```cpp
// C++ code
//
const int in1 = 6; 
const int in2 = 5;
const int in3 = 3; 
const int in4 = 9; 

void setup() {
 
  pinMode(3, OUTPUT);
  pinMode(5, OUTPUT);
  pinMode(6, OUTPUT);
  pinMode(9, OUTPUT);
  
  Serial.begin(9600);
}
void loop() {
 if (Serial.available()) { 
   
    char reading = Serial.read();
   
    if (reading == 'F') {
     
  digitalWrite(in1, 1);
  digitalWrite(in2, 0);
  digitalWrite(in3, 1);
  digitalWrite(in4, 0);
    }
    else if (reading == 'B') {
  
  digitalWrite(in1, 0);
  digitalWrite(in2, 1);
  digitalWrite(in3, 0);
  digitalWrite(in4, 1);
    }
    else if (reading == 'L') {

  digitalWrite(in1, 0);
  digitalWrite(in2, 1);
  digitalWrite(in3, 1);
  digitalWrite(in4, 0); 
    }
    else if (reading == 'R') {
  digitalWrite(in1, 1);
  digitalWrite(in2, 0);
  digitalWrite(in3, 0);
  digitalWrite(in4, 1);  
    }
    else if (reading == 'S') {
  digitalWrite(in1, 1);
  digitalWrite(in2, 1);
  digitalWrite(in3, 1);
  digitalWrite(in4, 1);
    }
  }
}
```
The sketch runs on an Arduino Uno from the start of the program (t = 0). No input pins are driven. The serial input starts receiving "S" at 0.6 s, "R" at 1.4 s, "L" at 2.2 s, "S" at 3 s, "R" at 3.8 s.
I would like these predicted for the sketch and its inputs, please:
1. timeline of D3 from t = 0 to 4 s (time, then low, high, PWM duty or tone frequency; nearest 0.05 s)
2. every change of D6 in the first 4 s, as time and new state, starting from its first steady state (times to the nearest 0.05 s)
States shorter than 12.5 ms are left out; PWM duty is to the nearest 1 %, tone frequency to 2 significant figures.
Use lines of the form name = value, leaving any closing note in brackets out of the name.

timeline of D3 from t = 0 to 4 s = 0 s low; 0.6 s high; 1.4 s low; 2.2 s high; 3.8 s low
every change of D6 in the first 4 s, as time and new state, starting from its first steady state = 0 s low; 0.6 s high; 2.2 s low; 3 s high
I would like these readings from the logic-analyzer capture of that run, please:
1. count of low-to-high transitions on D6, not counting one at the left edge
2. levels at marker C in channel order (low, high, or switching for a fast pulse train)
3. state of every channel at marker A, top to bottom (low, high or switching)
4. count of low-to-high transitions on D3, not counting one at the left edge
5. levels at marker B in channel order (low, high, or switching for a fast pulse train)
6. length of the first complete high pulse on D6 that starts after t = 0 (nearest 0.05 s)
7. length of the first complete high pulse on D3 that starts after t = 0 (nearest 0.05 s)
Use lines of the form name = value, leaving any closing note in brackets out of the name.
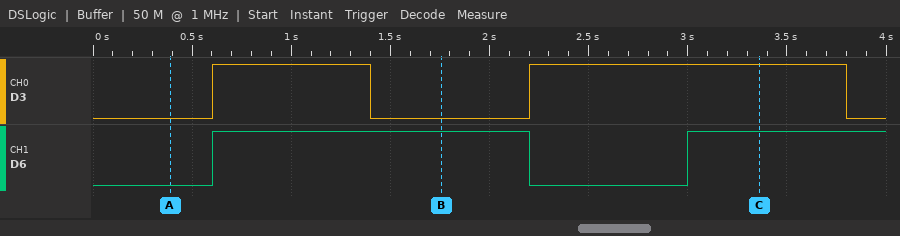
count of low-to-high transitions on D6, not counting one at the left edge = 2
levels at marker C in channel order = D3 high, D6 high
state of every channel at marker A, top to bottom = D3 low, D6 low
count of low-to-high transitions on D3, not counting one at the left edge = 2
levels at marker B in channel order = D3 low, D6 high
length of the first complete high pulse on D6 that starts after t = 0 = 1.60 s
length of the first complete high pulse on D3 that starts after t = 0 = 0.80 s
